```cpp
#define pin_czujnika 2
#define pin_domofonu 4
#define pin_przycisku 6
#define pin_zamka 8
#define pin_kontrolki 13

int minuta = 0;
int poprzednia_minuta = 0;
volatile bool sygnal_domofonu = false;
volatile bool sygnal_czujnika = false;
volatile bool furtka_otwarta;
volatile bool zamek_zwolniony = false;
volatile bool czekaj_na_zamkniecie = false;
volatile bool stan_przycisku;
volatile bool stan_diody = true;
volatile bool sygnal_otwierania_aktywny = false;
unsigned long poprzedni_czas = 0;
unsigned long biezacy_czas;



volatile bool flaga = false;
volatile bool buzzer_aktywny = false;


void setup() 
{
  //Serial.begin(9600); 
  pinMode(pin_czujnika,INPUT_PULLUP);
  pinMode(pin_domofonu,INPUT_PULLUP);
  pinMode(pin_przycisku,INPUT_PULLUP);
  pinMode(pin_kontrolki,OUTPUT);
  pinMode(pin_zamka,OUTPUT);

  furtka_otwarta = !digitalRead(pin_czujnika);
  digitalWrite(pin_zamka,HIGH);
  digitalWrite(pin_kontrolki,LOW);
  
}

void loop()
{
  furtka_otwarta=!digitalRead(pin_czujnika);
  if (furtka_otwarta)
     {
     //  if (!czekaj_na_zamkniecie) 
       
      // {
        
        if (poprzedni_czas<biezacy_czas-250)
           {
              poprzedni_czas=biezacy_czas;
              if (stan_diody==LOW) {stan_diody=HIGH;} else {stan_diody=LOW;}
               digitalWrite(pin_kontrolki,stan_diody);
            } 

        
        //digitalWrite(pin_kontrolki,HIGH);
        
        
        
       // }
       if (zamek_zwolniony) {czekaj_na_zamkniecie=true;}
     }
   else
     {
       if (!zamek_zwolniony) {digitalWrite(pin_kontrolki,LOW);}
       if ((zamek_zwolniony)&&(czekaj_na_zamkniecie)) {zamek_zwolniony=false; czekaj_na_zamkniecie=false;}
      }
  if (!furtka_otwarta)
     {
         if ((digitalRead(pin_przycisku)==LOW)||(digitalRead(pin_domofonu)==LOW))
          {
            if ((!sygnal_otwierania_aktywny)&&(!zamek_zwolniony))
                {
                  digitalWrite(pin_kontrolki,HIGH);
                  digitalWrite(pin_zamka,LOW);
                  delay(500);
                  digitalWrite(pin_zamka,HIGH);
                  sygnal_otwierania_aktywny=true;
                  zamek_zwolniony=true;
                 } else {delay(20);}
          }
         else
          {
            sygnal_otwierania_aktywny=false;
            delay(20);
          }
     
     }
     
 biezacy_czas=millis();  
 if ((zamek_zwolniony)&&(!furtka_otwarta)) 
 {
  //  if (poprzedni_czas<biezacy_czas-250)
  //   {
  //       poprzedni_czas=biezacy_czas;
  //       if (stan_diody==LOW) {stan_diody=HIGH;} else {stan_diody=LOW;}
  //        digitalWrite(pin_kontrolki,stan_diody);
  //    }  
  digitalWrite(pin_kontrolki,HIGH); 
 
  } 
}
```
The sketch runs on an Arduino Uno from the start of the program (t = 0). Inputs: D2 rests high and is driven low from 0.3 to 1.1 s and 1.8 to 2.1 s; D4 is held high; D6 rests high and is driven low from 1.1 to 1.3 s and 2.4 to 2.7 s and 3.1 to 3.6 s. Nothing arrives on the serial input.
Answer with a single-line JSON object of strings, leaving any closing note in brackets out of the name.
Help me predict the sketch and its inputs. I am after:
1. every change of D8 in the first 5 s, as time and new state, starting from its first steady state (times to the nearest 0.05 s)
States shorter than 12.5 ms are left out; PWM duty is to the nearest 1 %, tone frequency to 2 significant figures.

{"every change of D8 in the first 5 s, as time and new state, starting from its first steady state": "0 s high; 1.1 s low; 1.6 s high; 2.4 s low; 2.9 s high"}
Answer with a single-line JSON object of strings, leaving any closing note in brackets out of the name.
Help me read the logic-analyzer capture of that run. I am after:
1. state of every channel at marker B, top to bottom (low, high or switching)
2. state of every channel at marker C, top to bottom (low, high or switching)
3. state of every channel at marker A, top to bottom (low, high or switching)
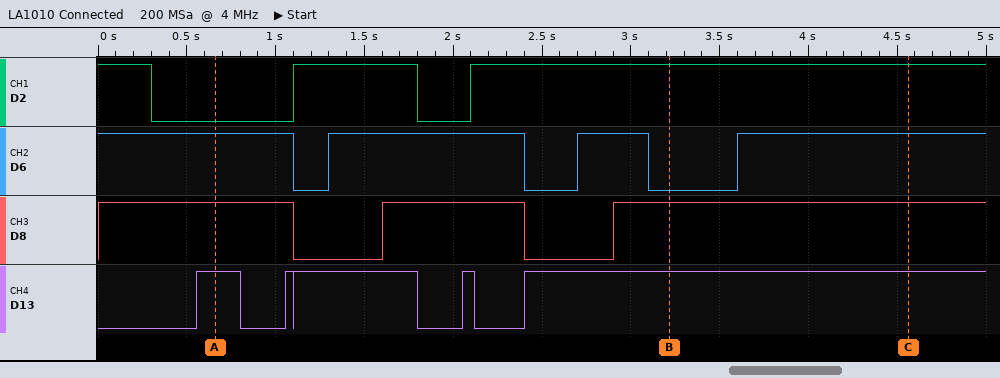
{"state of every channel at marker B, top to bottom": "D2 high, D6 low, D8 high, D13 high", "state of every channel at marker C, top to bottom": "D2 high, D6 high, D8 high, D13 high", "state of every channel at marker A, top to bottom": "D2 low, D6 high, D8 high, D13 high"}
